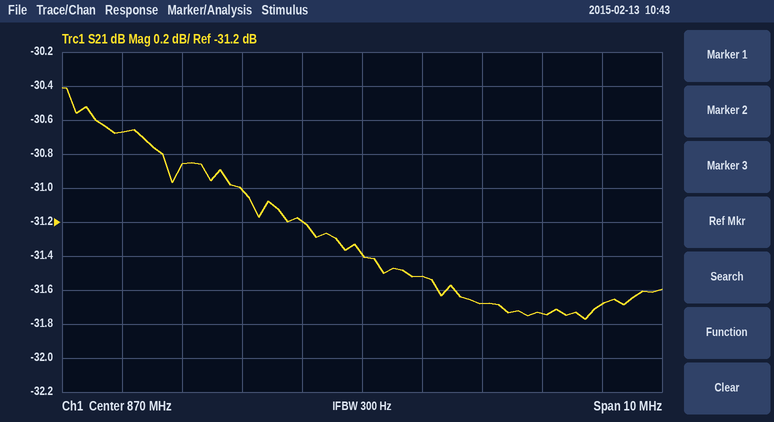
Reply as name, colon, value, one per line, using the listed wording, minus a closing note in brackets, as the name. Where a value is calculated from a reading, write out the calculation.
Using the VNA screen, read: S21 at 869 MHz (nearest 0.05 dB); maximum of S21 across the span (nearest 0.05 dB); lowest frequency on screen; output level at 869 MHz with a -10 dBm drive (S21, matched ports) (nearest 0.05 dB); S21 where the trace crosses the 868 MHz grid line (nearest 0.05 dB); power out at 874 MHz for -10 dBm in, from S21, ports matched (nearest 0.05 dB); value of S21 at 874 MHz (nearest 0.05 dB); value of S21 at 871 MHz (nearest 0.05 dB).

S21 at 869 MHz: -31.20 dB
maximum of S21 across the span: -30.40 dB
lowest frequency on screen: 865 MHz
output level at 869 MHz with a -10 dBm drive (S21, matched ports): -10 dBm + (-31.20 dB) = -41.20 dBm
S21 where the trace crosses the 868 MHz grid line: -31.00 dB
power out at 874 MHz for -10 dBm in, from S21, ports matched: -10 dBm + (-31.70 dB) = -41.70 dBm
value of S21 at 874 MHz: -31.70 dB
value of S21 at 871 MHz: -31.50 dB
